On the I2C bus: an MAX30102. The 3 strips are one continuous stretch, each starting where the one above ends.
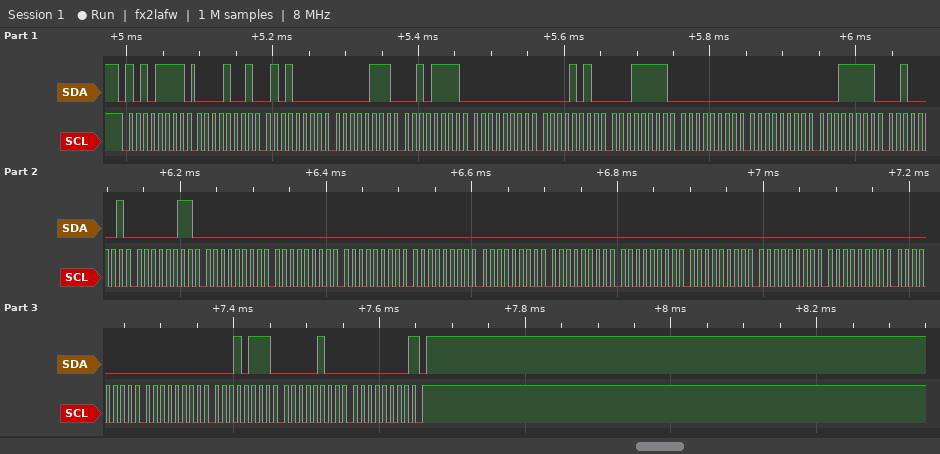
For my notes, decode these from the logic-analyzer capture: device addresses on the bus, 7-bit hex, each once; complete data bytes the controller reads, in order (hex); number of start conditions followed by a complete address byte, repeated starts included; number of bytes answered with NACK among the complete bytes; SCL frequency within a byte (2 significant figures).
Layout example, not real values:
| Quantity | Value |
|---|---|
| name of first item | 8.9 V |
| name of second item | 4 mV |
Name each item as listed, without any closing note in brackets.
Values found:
| Quantity | Value |
|---|---|
| device addresses on the bus, 7-bit hex, each once | 0x57 |
| complete data bytes the controller reads, in order | 09 50 07 2F 00 0A 1F 00 00 1F 21 03 00 00 00 00 00 00 00 00 00 00 00 00 17 04 00 |
| number of start conditions followed by a complete address byte, repeated starts included | 1 |
| number of bytes answered with NACK among the complete bytes | 1 |
| SCL frequency within a byte | 100 kHz |
